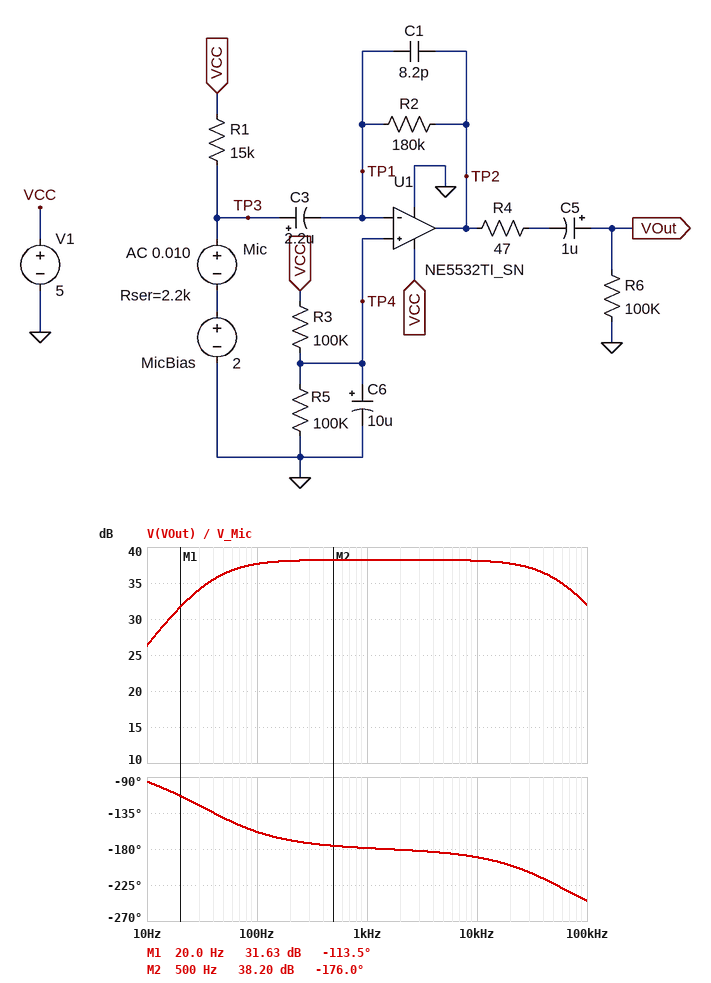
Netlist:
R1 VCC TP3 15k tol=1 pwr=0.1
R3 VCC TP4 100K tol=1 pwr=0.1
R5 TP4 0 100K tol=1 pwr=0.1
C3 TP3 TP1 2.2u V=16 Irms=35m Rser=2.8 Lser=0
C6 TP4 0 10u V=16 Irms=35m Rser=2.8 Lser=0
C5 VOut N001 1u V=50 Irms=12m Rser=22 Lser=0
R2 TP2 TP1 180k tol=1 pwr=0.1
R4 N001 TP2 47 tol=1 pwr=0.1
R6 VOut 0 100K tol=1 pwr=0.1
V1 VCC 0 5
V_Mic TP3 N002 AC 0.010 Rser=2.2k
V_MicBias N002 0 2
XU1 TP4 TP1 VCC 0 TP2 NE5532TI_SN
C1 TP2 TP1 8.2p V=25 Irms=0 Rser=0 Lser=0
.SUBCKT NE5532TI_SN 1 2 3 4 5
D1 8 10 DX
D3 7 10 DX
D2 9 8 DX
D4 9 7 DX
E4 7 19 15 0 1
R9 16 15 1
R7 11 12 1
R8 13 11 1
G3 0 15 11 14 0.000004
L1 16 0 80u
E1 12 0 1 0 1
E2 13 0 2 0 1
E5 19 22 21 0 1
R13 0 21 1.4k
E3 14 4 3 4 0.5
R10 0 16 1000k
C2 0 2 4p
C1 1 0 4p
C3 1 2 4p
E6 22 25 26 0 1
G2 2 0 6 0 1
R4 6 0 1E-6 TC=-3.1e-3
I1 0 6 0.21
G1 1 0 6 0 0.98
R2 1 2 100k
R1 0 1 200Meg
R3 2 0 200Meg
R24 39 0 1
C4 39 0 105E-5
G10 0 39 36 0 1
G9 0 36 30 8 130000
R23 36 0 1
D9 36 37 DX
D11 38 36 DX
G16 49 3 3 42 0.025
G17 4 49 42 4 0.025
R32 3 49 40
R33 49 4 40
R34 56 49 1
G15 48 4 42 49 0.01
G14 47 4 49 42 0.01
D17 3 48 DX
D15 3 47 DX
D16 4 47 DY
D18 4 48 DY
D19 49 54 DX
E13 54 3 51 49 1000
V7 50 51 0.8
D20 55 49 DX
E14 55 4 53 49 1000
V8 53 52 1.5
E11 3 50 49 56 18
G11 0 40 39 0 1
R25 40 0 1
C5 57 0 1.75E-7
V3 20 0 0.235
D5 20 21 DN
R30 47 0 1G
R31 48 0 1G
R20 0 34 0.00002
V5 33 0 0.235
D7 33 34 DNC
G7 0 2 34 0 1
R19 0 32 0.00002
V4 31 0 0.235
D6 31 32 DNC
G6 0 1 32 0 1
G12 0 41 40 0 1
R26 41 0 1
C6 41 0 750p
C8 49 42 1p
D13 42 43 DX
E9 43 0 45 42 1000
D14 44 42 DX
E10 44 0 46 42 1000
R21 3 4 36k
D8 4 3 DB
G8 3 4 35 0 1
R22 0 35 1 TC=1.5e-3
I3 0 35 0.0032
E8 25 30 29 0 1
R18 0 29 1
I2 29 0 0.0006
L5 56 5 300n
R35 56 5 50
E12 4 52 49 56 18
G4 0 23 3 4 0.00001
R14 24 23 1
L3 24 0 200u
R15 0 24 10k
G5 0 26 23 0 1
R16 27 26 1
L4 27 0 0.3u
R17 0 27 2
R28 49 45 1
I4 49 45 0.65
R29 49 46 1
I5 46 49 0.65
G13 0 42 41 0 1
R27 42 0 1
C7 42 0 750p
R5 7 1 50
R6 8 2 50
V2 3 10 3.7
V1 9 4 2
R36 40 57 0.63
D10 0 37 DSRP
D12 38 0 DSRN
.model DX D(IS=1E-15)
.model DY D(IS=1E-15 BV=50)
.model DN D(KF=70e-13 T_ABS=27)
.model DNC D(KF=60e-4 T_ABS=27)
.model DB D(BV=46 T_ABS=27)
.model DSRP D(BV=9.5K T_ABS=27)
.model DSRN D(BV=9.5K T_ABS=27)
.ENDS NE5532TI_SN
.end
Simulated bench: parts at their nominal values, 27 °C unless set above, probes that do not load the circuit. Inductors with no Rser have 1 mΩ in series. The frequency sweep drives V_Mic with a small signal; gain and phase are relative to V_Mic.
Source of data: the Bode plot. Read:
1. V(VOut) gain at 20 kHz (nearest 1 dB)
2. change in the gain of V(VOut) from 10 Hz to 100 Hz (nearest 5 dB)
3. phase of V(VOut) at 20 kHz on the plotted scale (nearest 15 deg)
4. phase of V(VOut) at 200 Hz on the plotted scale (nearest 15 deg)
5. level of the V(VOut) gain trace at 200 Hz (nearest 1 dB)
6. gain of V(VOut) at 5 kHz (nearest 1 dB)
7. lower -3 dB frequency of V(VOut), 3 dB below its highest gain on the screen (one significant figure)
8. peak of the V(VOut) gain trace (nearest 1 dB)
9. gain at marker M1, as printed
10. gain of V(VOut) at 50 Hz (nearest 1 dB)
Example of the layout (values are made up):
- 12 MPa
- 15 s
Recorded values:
- 38 dB
- 10 dB
- -195 deg
- -165 deg
- 38 dB
- 38 dB
- 40 Hz
- 38 dB
- 31.63 dB
- 36 dB
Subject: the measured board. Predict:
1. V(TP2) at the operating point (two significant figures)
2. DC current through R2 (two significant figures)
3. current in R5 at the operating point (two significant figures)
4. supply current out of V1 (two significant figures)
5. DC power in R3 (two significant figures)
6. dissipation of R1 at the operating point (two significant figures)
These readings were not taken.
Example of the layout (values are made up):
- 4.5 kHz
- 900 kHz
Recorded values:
- 4.1 V
- 12 µA
- 19 µA
- 3.5 mA
- 96 µW
- 460 µW
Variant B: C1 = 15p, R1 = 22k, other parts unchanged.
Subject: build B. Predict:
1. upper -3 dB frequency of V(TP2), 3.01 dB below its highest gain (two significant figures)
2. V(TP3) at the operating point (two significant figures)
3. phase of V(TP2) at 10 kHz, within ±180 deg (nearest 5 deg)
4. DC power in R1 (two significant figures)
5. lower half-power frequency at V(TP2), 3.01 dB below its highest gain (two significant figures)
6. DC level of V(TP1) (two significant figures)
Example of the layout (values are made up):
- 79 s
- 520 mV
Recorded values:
- 39 kHz
- 2.3 V
- 165 deg
- 340 µW
- 36 Hz
- 1.9 V
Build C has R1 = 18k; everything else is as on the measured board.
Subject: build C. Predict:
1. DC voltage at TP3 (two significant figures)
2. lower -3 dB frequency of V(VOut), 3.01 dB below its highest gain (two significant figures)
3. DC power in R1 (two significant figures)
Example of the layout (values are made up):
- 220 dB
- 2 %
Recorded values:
- 2.3 V
- 37 Hz
- 400 µW
